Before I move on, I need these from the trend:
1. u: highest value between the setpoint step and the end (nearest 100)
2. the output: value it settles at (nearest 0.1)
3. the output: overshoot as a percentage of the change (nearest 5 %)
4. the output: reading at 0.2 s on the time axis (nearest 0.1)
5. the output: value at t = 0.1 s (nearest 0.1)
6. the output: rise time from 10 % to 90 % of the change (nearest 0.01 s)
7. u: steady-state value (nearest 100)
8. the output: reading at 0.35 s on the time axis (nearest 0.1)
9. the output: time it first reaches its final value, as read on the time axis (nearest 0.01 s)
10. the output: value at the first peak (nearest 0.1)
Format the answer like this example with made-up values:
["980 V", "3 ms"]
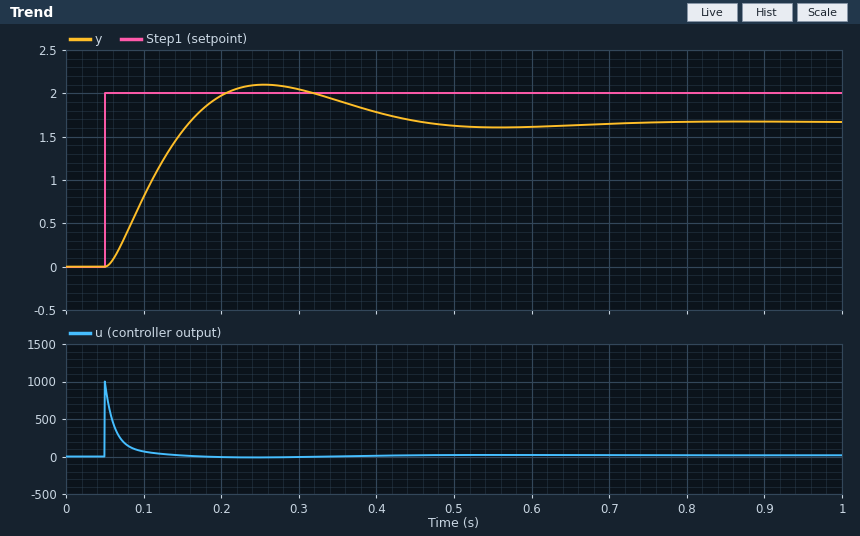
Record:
["1000", "1.7", "25 %", "2.0", "0.8", "0.08 s", "0", "1.9", "0.16 s", "2.1"]
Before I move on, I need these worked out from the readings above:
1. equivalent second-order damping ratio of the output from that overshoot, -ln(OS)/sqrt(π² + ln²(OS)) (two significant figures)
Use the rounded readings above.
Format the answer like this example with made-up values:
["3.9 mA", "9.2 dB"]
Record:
["0.40"]
